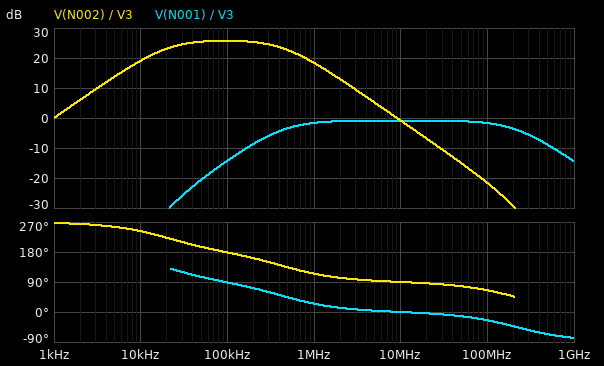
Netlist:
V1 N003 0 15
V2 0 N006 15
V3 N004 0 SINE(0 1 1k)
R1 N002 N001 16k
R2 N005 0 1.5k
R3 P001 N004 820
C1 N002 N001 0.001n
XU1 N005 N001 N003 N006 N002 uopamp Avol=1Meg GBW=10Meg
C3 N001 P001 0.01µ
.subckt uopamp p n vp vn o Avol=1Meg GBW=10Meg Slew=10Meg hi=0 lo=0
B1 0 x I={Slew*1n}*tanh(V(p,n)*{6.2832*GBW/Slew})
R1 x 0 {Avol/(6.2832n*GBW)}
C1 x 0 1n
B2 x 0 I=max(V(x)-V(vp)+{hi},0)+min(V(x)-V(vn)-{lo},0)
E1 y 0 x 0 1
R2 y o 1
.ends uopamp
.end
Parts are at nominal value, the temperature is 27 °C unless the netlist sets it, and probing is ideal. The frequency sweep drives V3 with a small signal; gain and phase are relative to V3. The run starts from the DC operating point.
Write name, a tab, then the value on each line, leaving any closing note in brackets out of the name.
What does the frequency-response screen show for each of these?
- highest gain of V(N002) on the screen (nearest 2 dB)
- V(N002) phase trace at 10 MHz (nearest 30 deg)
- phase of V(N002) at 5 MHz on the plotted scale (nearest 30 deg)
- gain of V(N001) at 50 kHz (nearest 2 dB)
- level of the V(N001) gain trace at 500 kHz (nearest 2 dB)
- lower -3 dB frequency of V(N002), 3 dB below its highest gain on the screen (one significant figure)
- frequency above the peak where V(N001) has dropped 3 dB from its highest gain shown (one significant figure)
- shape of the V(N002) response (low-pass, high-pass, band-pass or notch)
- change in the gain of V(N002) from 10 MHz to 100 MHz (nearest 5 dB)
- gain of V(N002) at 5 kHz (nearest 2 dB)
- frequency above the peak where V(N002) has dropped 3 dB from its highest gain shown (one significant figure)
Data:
highest gain of V(N002) on the screen	26 dB
V(N002) phase trace at 10 MHz	90 deg
phase of V(N002) at 5 MHz on the plotted scale	90 deg
gain of V(N001) at 50 kHz	-20 dB
level of the V(N001) gain trace at 500 kHz	-4 dB
lower -3 dB frequency of V(N002), 3 dB below its highest gain on the screen	20 kHz
frequency above the peak where V(N001) has dropped 3 dB from its highest gain shown	200 MHz
shape of the V(N002) response	band-pass
change in the gain of V(N002) from 10 MHz to 100 MHz	-20 dB
gain of V(N002) at 5 kHz	14 dB
frequency above the peak where V(N002) has dropped 3 dB from its highest gain shown	500 kHz
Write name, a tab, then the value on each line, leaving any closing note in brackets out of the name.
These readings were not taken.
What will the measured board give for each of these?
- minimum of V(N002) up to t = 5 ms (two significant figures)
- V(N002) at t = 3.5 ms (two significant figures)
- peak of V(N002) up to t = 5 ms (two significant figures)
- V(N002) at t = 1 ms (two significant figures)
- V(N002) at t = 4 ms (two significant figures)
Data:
minimum of V(N002) up to t = 5 ms	-1.0 V
V(N002) at t = 3.5 ms	1.0 V
peak of V(N002) up to t = 5 ms	1.0 V
V(N002) at t = 1 ms	-1.0 V
V(N002) at t = 4 ms	-1.0 V
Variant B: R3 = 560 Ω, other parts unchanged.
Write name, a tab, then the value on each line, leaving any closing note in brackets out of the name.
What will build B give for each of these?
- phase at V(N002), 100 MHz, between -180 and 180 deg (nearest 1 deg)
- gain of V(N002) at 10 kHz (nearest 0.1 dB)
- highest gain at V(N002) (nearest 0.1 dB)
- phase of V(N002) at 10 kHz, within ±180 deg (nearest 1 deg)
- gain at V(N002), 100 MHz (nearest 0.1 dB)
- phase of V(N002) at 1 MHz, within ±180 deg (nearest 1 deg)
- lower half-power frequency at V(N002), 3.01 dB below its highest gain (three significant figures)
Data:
phase at V(N002), 100 MHz, between -180 and 180 deg	72 deg
gain of V(N002) at 10 kHz	19.6 dB
highest gain at V(N002)	29.1 dB
phase of V(N002) at 10 kHz, within ±180 deg	-110 deg
gain at V(N002), 100 MHz	-21.0 dB
phase of V(N002) at 1 MHz, within ±180 deg	108 deg
lower half-power frequency at V(N002), 3.01 dB below its highest gain	26.2 kHz
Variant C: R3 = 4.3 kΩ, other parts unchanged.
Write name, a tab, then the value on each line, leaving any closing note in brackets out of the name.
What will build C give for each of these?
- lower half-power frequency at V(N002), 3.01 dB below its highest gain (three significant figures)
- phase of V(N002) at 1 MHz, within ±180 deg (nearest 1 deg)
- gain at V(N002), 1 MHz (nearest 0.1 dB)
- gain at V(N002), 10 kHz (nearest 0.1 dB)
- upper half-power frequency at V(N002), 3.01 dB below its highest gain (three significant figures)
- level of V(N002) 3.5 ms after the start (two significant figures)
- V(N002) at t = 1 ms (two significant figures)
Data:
lower half-power frequency at V(N002), 3.01 dB below its highest gain	3.69 kHz
phase of V(N002) at 1 MHz, within ±180 deg	150 deg
gain at V(N002), 1 MHz	10.3 dB
gain at V(N002), 10 kHz	10.9 dB
upper half-power frequency at V(N002), 3.01 dB below its highest gain	1.81 MHz
level of V(N002) 3.5 ms after the start	940 mV
V(N002) at t = 1 ms	-940 mV
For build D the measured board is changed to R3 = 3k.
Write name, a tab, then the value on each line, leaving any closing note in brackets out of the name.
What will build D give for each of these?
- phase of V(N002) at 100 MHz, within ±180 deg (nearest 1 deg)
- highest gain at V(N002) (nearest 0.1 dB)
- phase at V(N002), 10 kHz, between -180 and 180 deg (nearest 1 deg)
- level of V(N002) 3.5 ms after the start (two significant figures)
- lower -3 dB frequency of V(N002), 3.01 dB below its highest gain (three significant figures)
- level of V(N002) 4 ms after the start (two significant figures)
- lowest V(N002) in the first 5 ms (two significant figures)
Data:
phase of V(N002) at 100 MHz, within ±180 deg	36 deg
highest gain at V(N002)	14.5 dB
phase at V(N002), 10 kHz, between -180 and 180 deg	-152 deg
level of V(N002) 3.5 ms after the start	970 mV
lower -3 dB frequency of V(N002), 3.01 dB below its highest gain	5.28 kHz
level of V(N002) 4 ms after the start	-970 mV
lowest V(N002) in the first 5 ms	-990 mV
